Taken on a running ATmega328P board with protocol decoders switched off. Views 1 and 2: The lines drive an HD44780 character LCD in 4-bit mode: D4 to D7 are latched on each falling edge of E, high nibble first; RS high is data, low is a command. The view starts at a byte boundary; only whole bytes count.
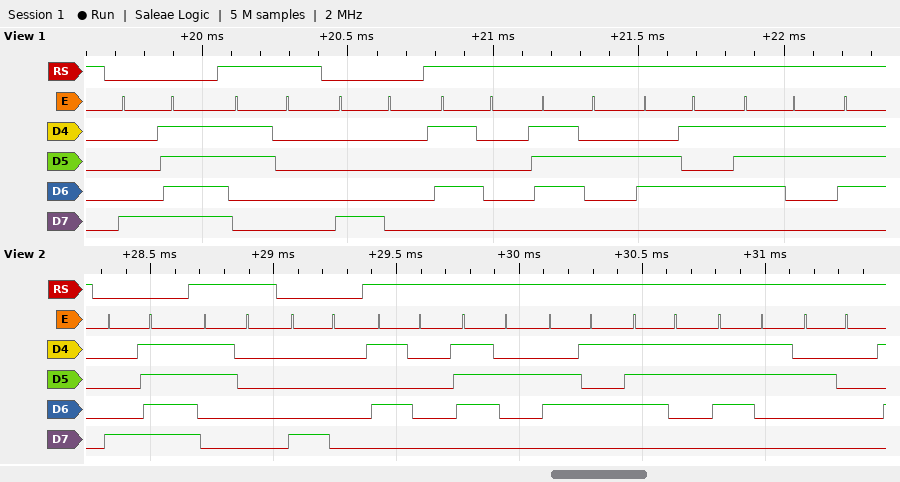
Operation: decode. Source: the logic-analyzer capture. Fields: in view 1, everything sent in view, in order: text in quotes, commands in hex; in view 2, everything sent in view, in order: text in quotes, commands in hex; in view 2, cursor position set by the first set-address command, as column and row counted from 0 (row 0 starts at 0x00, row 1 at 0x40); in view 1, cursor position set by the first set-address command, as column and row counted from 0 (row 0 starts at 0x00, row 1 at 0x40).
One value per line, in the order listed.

0x8F "0" 0x80 "Pres"
0x8F "0" 0x80 "Press "
column 15, row 0
column 15, row 0
